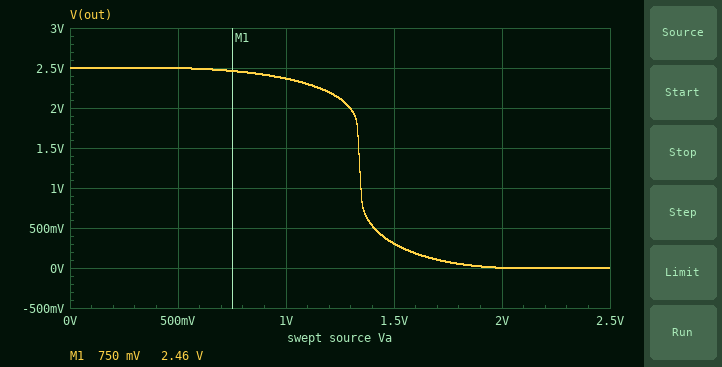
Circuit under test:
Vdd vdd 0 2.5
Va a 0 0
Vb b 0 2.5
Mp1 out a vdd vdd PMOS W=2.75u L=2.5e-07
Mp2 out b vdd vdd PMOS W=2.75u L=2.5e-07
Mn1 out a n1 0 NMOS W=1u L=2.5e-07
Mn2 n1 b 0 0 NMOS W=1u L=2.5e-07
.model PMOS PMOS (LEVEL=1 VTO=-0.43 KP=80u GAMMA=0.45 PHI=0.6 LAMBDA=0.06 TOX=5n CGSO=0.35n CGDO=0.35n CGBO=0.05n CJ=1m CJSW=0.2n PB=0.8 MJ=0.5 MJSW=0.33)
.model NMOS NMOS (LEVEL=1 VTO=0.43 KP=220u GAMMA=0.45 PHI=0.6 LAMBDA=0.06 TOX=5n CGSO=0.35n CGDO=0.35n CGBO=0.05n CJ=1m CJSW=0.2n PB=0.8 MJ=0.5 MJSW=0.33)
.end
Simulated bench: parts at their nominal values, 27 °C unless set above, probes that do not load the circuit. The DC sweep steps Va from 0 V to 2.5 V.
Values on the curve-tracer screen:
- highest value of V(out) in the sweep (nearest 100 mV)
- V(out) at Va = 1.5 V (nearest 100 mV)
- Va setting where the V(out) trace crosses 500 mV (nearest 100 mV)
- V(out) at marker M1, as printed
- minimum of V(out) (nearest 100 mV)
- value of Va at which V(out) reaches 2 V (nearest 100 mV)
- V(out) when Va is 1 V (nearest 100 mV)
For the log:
2.5 V
300 mV
1.4 V
2.46 V
0 V
1.3 V
2.4 V
